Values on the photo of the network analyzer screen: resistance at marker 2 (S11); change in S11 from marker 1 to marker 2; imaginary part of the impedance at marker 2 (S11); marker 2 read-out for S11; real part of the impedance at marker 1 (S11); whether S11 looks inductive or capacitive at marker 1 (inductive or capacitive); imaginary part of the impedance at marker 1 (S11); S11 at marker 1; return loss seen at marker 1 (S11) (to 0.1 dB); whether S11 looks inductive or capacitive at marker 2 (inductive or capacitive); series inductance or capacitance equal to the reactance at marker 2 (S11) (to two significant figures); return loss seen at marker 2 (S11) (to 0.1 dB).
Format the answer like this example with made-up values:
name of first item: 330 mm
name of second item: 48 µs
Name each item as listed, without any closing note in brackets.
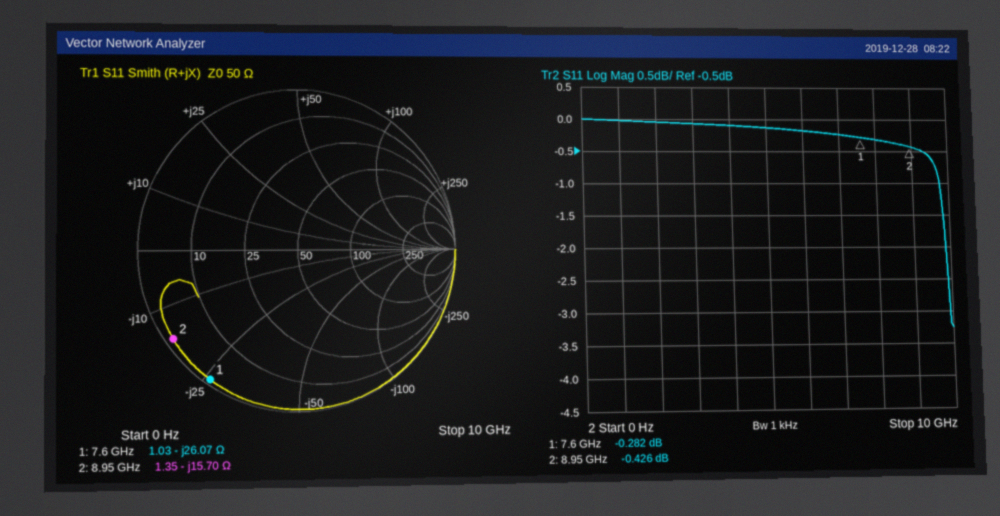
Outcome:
resistance at marker 2: 1.35 Ω
change in S11 from marker 1 to marker 2: -0.144 dB
imaginary part of the impedance at marker 2: -15.70 Ω
marker 2 read-out for S11: -0.426 dB
real part of the impedance at marker 1: 1.03 Ω
whether S11 looks inductive or capacitive at marker 1: capacitive
imaginary part of the impedance at marker 1: -26.07 Ω
S11 at marker 1: -0.282 dB
return loss seen at marker 1 (S11): 0.3 dB
whether S11 looks inductive or capacitive at marker 2: capacitive
series inductance or capacitance equal to the reactance at marker 2 (S11): 1.1 pF
return loss seen at marker 2 (S11): 0.4 dB
